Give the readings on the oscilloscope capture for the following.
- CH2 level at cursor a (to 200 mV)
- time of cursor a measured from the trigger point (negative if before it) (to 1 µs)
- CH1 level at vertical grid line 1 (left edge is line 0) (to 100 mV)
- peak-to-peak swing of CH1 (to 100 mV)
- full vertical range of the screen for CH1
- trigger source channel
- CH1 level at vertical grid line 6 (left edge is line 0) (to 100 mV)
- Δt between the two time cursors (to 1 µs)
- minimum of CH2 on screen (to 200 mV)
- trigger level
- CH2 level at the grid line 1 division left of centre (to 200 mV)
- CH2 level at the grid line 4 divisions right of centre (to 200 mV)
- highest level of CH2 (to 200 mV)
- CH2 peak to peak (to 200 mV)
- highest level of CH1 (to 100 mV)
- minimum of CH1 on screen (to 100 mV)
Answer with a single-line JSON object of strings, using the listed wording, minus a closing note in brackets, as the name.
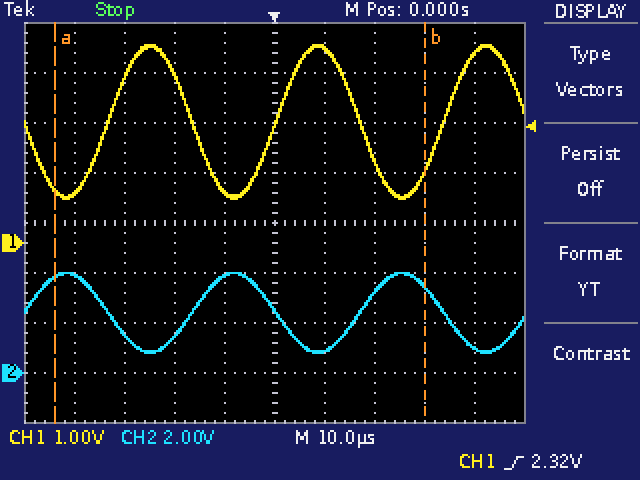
{"CH2 level at cursor a": "3.8 V", "time of cursor a measured from the trigger point (negative if before it)": "-44 µs", "CH1 level at vertical grid line 1 (left edge is line 0)": "1.0 V", "peak-to-peak swing of CH1": "3.1 V", "full vertical range of the screen for CH1": "8 V", "trigger source channel": "CH1", "CH1 level at vertical grid line 6 (left edge is line 0)": "3.9 V", "Δt between the two time cursors": "74 µs", "minimum of CH2 on screen": "800 mV", "trigger level": "2.32 V", "CH2 level at the grid line 1 division left of centre": "3.8 V", "CH2 level at the grid line 4 divisions right of centre": "1.0 V", "highest level of CH2": "4.0 V", "CH2 peak to peak": "3.2 V", "highest level of CH1": "4.0 V", "minimum of CH1 on screen": "900 mV"}
